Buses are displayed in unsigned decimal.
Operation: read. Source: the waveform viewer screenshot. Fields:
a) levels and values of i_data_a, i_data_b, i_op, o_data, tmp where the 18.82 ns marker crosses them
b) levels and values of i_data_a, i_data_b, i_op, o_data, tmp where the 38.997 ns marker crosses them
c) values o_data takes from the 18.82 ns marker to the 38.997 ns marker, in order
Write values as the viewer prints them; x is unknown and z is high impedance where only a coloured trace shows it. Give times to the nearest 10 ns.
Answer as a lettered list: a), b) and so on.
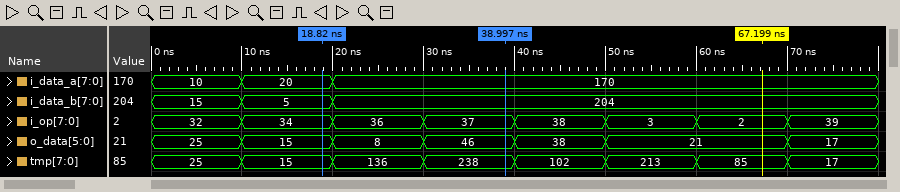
a) i_data_a=20, i_data_b=5, i_op=34, o_data=15, tmp=15
b) i_data_a=170, i_data_b=204, i_op=37, o_data=46, tmp=238
c) 15, 8, 46
